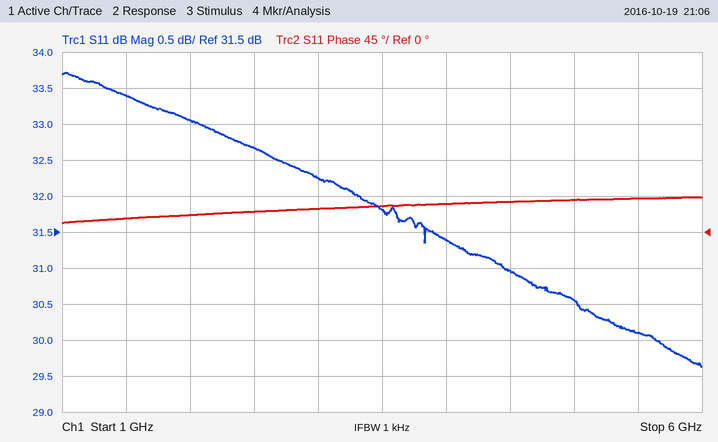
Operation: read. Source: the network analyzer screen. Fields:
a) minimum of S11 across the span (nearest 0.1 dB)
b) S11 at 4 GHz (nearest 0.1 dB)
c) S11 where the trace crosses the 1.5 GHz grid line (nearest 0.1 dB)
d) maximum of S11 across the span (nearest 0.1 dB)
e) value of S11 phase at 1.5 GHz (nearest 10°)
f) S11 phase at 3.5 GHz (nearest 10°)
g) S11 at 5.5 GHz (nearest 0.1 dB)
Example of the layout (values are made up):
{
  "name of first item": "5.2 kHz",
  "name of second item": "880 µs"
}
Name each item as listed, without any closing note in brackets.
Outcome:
{
  "minimum of S11 across the span": "29.6 dB",
  "S11 at 4 GHz": "31.4 dB",
  "S11 where the trace crosses the 1.5 GHz grid line": "33.4 dB",
  "maximum of S11 across the span": "33.7 dB",
  "value of S11 phase at 1.5 GHz": "20°",
  "S11 phase at 3.5 GHz": "30°",
  "S11 at 5.5 GHz": "30.1 dB"
}
